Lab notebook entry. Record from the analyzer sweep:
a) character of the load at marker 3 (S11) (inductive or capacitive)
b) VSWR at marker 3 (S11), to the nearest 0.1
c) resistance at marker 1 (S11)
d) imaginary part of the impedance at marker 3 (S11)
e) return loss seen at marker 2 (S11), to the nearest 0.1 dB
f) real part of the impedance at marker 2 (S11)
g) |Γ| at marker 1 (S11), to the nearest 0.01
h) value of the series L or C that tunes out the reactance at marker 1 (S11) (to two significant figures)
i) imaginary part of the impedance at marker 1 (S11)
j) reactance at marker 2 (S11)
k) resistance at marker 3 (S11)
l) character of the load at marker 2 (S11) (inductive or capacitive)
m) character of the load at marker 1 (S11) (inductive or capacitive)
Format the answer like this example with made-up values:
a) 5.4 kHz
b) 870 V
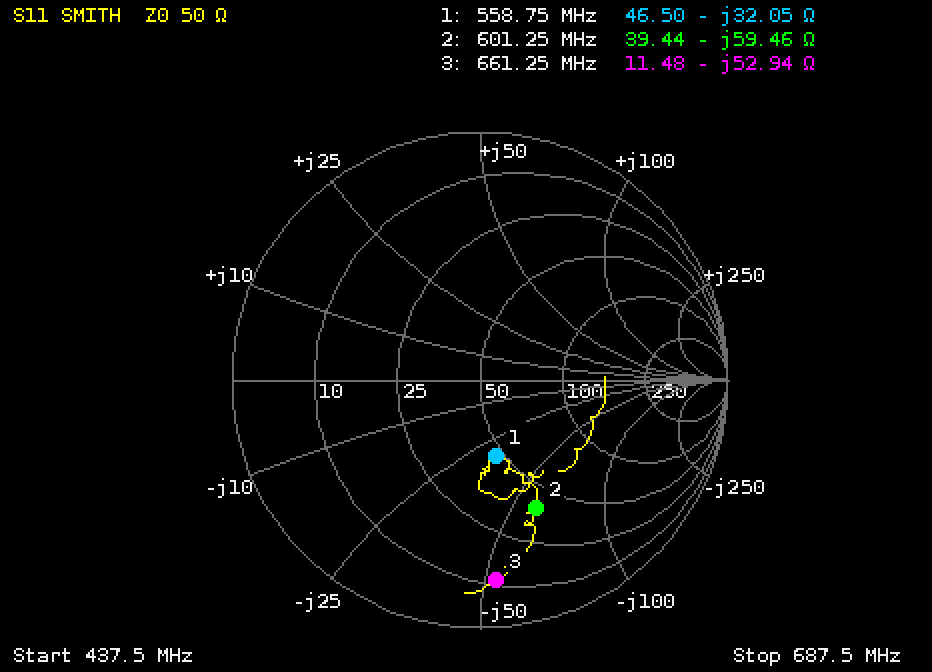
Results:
a) capacitive
b) 9.4
c) 46.50 Ω
d) -52.94 Ω
e) 5.0 dB
f) 39.44 Ω
g) 0.32
h) 9.1 nH
i) -32.05 Ω
j) -59.46 Ω
k) 11.48 Ω
l) capacitive
m) capacitive
